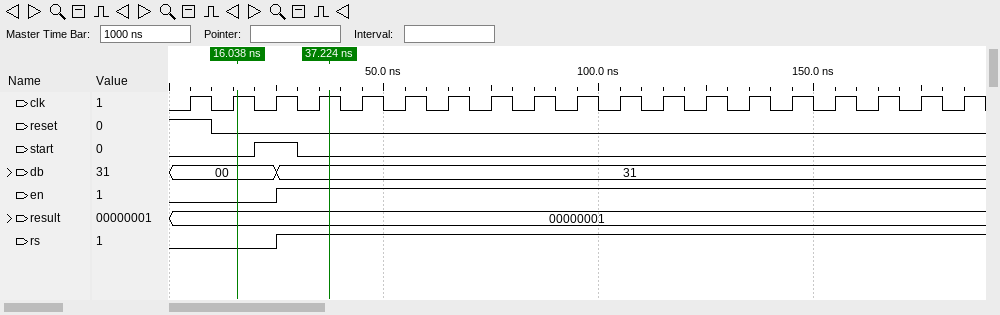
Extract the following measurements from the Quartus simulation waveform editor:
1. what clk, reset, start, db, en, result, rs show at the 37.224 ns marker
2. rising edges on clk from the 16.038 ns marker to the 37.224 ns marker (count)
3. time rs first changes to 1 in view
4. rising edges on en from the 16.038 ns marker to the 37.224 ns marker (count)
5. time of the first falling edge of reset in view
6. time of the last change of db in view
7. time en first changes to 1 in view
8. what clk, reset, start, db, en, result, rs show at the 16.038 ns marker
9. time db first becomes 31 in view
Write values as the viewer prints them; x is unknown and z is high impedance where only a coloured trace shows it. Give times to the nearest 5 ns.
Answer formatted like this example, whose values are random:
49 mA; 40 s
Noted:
clk=1, reset=0, start=0, db=31, en=1, result=00000001, rs=1; 2; 25 ns; 1; 10 ns; 25 ns; 25 ns; clk=1, reset=0, start=0, db=00, en=0, result=00000001, rs=0; 25 ns
